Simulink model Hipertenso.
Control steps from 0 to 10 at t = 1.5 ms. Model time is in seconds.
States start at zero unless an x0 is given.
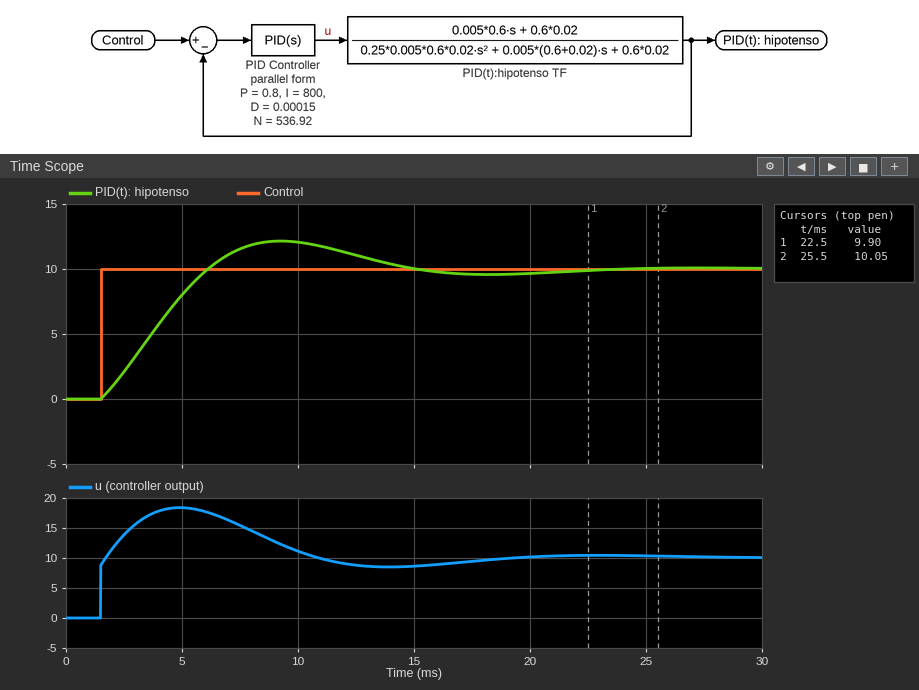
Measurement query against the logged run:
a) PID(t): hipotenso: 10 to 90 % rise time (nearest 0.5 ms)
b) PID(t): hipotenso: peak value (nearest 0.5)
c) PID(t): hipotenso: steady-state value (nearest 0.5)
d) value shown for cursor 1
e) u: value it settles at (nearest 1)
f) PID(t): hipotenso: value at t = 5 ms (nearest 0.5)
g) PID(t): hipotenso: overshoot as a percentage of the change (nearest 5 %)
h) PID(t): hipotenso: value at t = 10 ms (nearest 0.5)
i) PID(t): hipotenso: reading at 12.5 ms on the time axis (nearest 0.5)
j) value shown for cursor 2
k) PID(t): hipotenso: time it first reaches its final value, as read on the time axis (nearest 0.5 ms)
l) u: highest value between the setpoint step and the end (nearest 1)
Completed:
3.5 ms
12.0
10.0
9.90
10
8.0
20 %
12.0
11.0
10.05
6.0 ms
18
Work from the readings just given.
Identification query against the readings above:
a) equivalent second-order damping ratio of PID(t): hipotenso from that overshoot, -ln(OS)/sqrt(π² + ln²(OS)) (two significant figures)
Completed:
0.46
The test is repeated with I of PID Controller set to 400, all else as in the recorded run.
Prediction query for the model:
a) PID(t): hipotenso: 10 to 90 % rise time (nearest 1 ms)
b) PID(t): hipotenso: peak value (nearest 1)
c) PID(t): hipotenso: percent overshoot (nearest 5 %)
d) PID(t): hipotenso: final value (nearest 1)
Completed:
6 ms
11
10 %
10
